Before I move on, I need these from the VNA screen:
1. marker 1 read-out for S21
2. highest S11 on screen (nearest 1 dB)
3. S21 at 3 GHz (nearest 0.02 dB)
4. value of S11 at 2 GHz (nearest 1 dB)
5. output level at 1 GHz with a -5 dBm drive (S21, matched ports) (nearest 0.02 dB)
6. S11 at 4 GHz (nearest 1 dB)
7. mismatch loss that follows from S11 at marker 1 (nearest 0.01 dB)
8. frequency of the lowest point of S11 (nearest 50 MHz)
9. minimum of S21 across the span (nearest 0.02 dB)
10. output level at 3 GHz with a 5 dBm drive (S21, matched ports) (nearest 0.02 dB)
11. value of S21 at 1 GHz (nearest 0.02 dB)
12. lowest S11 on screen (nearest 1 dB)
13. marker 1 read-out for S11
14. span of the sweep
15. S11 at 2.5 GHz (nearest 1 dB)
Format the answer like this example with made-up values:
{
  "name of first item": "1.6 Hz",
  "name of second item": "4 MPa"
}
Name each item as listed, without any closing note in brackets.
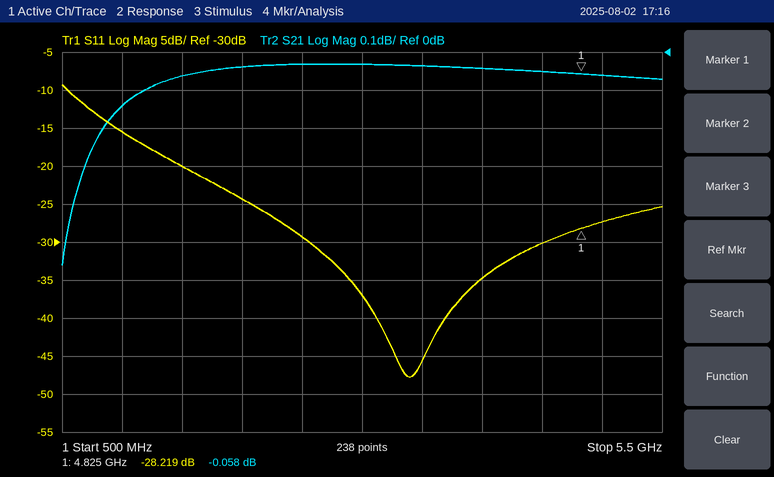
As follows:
{
  "marker 1 read-out for S21": "-0.058 dB",
  "highest S11 on screen": "-9 dB",
  "S21 at 3 GHz": "-0.04 dB",
  "value of S11 at 2 GHz": "-24 dB",
  "output level at 1 GHz with a -5 dBm drive (S21, matched ports)": "-5.14 dBm",
  "S11 at 4 GHz": "-35 dB",
  "mismatch loss that follows from S11 at marker 1": "0.01 dB",
  "frequency of the lowest point of S11": "3.40 GHz",
  "minimum of S21 across the span": "-0.56 dB",
  "output level at 3 GHz with a 5 dBm drive (S21, matched ports)": "4.96 dBm",
  "value of S21 at 1 GHz": "-0.14 dB",
  "lowest S11 on screen": "-48 dB",
  "marker 1 read-out for S11": "-28.219 dB",
  "span of the sweep": "5 GHz",
  "S11 at 2.5 GHz": "-29 dB"
}
